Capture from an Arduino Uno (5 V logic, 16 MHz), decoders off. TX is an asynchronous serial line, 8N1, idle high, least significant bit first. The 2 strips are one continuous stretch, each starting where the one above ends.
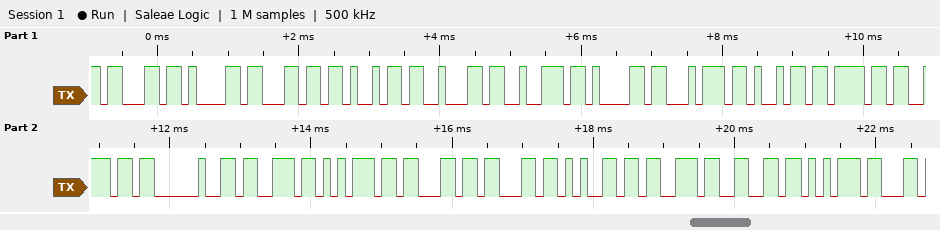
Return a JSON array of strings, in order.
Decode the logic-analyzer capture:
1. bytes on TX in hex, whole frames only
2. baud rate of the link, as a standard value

["63 61 6C 69 62 72 61 74 69 6F 6E 20 73 75 63 63 65 73 66 75", "9600 baud"]
